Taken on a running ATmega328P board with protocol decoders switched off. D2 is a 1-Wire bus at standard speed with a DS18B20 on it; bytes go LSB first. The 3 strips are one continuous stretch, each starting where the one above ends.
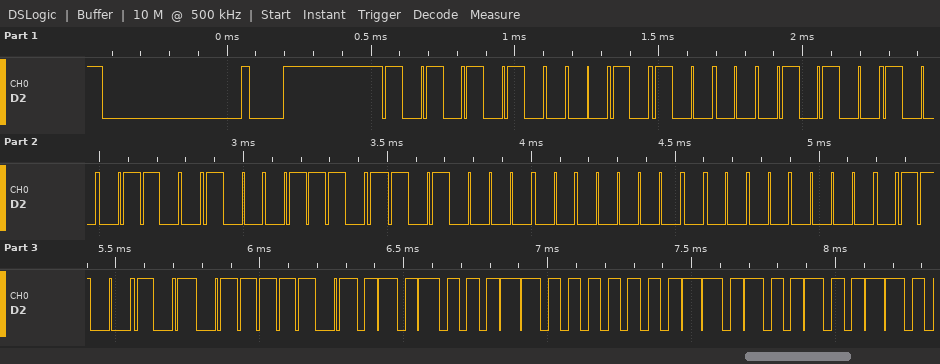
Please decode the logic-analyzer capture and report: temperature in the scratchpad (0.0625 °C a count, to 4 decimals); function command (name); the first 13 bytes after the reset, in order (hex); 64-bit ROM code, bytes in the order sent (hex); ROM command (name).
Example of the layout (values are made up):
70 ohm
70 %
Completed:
24.6250 °C
Read Scratchpad
55 28 28 31 71 0B 00 00 A6 BE 8A 01 4B
28 28 31 71 0B 00 00 A6
Match ROM
